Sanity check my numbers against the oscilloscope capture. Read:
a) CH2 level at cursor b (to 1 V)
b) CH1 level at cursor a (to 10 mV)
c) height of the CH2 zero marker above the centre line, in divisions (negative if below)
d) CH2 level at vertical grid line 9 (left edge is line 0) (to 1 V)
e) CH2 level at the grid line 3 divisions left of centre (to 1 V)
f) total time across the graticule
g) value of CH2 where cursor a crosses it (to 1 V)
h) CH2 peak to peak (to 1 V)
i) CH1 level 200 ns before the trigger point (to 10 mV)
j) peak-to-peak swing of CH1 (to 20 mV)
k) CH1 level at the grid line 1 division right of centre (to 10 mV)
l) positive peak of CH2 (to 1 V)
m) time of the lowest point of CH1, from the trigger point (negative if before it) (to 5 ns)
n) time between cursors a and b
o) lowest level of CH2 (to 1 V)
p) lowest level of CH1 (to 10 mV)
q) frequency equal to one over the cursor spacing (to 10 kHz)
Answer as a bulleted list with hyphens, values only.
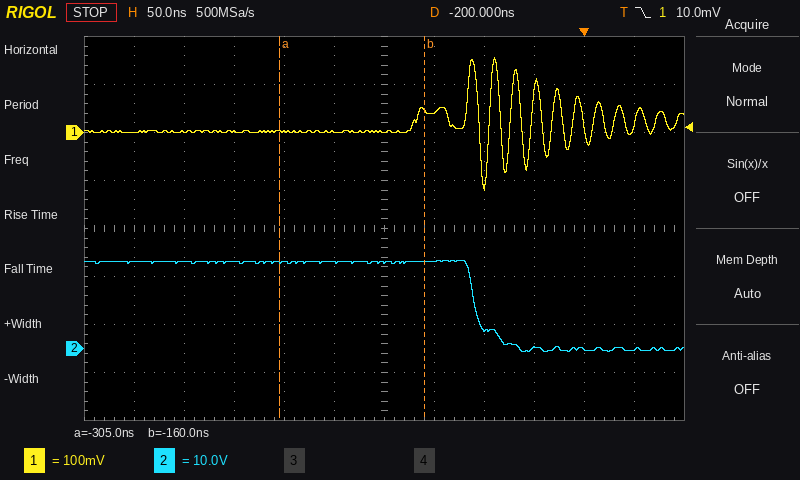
- 18 V
- 0 mV
- -2.5 div
- 0 V
- 18 V
- 600 ns
- 18 V
- 19 V
- 0 mV
- 280 mV
- 40 mV
- 18 V
- -100 ns
- 145 ns
- -1 V
- -120 mV
- 6.90 MHz
